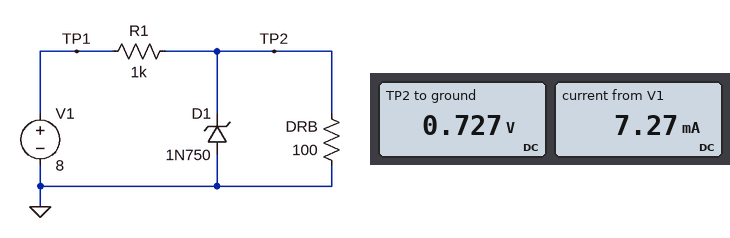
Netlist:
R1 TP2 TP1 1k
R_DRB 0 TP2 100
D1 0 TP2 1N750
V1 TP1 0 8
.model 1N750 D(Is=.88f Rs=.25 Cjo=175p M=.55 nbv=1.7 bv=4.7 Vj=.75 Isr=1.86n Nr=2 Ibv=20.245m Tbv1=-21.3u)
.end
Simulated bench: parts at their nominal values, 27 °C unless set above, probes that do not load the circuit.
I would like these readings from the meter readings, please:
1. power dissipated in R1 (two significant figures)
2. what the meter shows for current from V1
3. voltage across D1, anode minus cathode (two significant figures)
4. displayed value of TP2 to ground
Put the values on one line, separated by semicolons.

53 mW; 7.27 mA; -730 mV; 0.727 V
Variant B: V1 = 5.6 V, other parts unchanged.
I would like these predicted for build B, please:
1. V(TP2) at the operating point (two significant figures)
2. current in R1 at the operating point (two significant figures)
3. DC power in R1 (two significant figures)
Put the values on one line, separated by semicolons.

510 mV; 5.1 mA; 26 mW
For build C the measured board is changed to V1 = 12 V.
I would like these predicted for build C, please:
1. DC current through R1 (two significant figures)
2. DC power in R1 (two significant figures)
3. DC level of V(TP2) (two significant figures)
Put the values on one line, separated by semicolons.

11 mA; 120 mW; 1.1 V
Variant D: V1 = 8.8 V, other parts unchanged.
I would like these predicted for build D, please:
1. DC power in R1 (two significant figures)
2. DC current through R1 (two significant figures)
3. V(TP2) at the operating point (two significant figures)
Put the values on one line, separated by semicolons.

64 mW; 8.0 mA; 800 mV
